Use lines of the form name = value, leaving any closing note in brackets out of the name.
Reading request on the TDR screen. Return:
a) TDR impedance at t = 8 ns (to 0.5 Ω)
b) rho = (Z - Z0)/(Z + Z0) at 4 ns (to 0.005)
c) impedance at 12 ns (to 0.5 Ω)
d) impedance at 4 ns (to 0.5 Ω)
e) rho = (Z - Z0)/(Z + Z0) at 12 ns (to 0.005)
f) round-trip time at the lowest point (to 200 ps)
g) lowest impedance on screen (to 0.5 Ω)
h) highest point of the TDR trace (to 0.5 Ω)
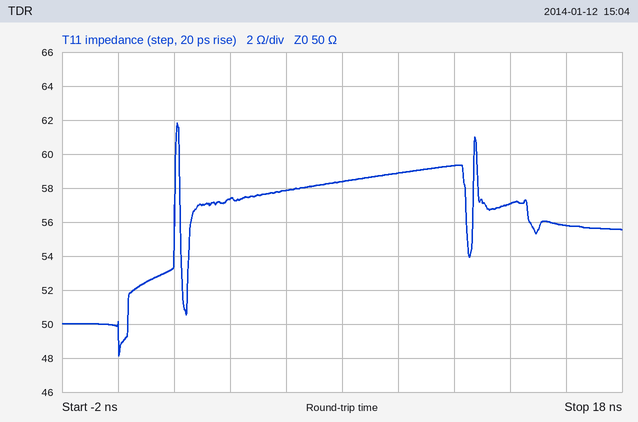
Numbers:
TDR impedance at t = 8 ns = 58.5 Ω
rho = (Z - Z0)/(Z + Z0) at 4 ns = +0.070
impedance at 12 ns = 59.5 Ω
impedance at 4 ns = 57.5 Ω
rho = (Z - Z0)/(Z + Z0) at 12 ns = +0.085
round-trip time at the lowest point = 0.0 ns
lowest impedance on screen = 48.0 Ω
highest point of the TDR trace = 62.0 Ω
